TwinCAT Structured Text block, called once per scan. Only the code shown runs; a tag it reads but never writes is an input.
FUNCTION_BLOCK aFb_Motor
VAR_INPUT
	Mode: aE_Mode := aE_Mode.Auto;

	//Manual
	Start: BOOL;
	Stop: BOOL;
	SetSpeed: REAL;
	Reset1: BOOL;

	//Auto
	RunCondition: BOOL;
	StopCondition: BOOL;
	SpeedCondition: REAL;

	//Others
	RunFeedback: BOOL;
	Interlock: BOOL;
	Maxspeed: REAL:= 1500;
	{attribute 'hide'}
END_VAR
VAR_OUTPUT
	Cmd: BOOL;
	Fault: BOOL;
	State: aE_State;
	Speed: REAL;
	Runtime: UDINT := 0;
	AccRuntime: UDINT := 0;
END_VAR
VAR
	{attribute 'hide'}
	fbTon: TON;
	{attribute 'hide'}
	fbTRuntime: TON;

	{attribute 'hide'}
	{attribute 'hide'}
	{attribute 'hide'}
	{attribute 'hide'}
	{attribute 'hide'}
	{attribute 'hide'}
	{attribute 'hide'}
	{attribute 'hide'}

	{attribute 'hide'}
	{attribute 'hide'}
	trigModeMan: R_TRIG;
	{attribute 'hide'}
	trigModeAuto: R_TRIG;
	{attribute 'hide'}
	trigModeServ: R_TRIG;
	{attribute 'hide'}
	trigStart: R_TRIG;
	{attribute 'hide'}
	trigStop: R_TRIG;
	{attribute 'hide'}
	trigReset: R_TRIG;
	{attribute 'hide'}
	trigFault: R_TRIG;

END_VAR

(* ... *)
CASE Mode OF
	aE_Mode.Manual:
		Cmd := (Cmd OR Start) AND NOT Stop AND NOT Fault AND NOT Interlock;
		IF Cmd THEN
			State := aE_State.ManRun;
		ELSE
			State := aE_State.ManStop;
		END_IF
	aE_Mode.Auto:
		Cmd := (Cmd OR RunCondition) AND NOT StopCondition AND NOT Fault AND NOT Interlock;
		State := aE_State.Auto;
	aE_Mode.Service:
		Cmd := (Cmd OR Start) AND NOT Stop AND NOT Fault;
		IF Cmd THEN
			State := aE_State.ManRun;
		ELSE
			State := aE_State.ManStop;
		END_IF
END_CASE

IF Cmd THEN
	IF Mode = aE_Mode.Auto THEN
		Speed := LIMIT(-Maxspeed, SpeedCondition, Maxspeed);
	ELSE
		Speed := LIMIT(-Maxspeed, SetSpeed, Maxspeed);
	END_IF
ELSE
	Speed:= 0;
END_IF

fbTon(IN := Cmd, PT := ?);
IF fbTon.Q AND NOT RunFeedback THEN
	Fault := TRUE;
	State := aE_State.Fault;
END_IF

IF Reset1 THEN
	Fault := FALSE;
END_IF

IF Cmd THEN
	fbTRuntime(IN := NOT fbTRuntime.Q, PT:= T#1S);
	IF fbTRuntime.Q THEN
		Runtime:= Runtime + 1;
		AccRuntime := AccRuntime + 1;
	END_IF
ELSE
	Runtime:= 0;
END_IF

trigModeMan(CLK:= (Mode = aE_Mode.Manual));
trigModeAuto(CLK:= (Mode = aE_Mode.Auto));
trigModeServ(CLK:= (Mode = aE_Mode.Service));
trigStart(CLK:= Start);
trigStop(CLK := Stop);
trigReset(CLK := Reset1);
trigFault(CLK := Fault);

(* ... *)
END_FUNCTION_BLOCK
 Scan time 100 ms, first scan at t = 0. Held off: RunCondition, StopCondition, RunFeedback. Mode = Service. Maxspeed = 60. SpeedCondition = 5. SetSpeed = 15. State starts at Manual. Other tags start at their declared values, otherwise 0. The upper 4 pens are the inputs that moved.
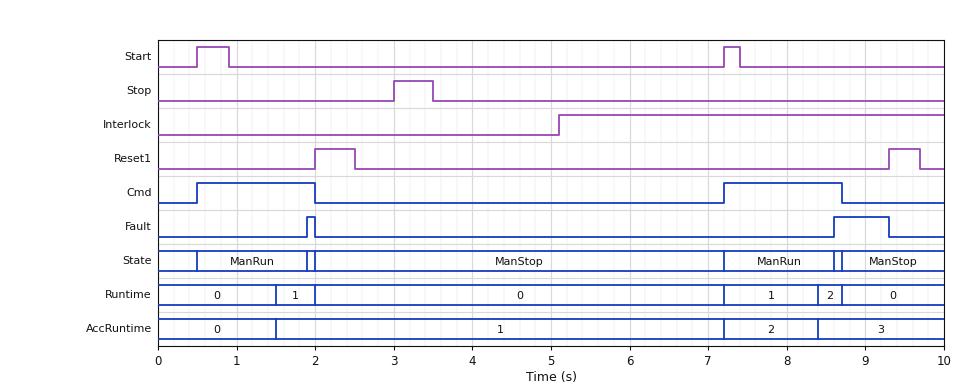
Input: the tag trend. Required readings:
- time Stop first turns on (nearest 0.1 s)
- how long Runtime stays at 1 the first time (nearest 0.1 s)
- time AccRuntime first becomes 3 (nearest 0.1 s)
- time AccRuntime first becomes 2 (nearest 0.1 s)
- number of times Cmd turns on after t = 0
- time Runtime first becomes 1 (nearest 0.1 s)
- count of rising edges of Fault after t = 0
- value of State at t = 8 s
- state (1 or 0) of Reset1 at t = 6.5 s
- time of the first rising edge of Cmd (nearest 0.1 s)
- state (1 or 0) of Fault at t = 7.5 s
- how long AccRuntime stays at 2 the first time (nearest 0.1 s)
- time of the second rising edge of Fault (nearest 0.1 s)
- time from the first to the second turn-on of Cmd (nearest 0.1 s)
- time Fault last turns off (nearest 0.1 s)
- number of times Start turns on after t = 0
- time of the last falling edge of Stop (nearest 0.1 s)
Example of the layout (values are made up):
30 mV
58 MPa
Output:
3.0 s
0.5 s
8.4 s
7.2 s
2
1.5 s
2
ManRun
0
0.5 s
0
1.2 s
8.6 s
6.7 s
9.3 s
2
3.5 s
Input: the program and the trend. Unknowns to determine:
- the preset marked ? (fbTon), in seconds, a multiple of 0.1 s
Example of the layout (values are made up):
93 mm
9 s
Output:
1.4 s
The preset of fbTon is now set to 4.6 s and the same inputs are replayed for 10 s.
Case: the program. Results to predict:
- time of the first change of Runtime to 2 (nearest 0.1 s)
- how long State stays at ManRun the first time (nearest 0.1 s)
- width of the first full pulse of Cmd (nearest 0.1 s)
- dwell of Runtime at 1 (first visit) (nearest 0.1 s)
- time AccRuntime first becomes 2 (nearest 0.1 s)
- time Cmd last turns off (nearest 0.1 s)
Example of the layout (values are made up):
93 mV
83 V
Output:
2.7 s
2.5 s
2.5 s
1.2 s
2.7 s
3.0 s
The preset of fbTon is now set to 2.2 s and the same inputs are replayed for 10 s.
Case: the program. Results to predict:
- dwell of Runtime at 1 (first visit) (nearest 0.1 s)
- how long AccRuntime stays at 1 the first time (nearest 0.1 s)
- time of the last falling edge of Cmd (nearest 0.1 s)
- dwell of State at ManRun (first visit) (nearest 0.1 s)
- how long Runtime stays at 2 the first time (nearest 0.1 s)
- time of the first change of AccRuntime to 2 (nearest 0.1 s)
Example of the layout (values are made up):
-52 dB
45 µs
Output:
1.2 s
1.2 s
2.8 s
2.2 s
0.1 s
2.7 s
